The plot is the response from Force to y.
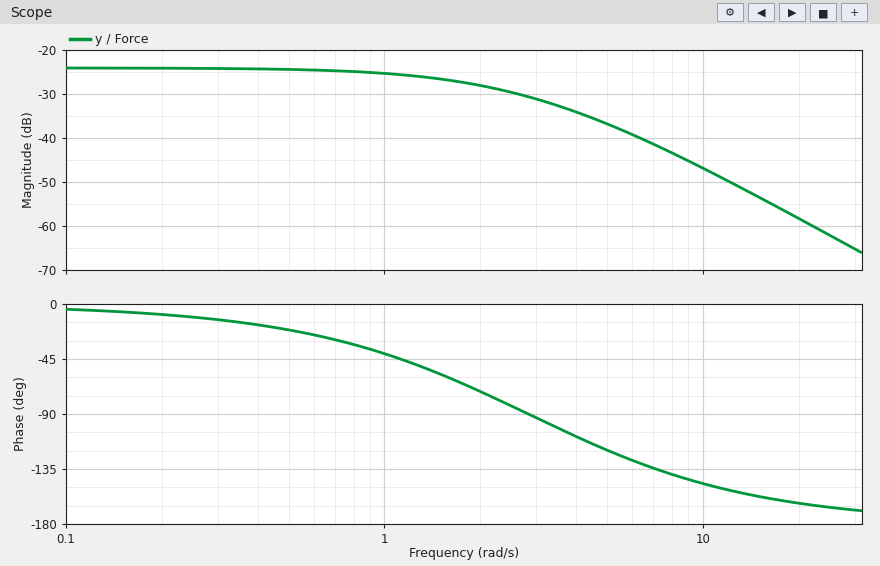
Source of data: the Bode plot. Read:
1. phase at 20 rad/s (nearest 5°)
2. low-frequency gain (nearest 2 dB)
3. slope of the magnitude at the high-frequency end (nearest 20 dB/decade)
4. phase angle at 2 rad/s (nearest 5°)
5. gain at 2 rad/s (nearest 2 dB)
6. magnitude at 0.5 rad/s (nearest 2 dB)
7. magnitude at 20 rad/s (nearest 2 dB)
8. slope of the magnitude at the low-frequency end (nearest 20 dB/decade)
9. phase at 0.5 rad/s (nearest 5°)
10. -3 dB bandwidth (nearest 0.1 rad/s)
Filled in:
-165°
-24 dB
-40 dB/decade
-70°
-28 dB
-24 dB
-58 dB
0 dB/decade
-20°
1.7 rad/s
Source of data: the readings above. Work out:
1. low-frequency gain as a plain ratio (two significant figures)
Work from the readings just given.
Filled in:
0.063
